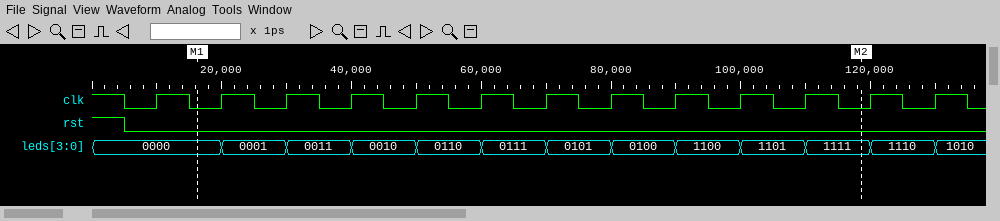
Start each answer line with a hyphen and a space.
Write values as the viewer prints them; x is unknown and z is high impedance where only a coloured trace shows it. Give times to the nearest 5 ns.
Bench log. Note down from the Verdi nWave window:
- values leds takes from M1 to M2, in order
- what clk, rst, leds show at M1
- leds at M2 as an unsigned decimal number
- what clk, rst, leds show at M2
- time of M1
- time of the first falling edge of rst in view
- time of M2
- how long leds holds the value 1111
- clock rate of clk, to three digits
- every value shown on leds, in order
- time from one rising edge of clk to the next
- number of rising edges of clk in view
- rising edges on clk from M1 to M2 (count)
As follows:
- 0000, 0001, 0011, 0010, 0110, 0111, 0101, 0100, 1100, 1101, 1111
- clk=0, rst=0, leds=0000
- 15
- clk=0, rst=0, leds=1111
- 15 ns
- 5 ns
- 120 ns
- 10 ns
- 100 MHz
- 0000, 0001, 0011, 0010, 0110, 0111, 0101, 0100, 1100, 1101, 1111, 1110, 1010
- 10 ns
- 13
- 10
